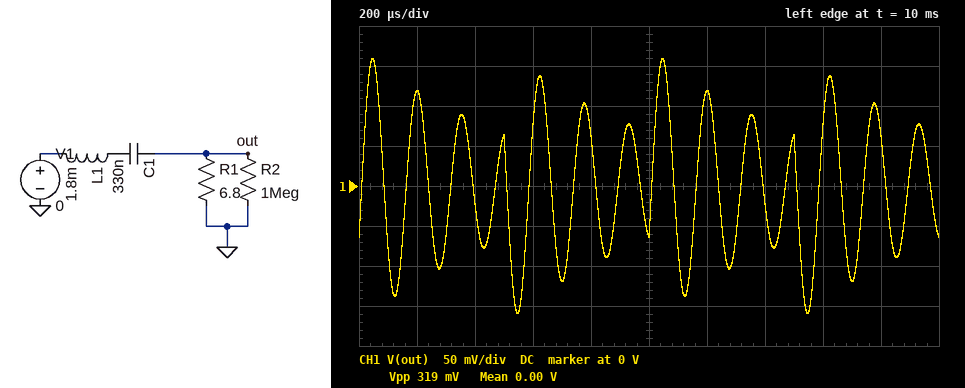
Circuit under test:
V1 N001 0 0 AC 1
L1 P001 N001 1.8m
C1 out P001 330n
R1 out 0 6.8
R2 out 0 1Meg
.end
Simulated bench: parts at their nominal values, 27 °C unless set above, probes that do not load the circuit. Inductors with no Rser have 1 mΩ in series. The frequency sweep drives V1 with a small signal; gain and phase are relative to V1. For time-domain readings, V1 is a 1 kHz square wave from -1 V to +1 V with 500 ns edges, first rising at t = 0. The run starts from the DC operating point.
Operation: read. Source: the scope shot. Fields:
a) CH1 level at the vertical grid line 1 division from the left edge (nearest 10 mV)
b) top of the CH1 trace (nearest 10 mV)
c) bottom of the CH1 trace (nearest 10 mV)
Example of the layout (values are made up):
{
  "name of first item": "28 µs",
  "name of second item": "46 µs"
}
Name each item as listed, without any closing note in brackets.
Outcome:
{
  "CH1 level at the vertical grid line 1 division from the left edge": "120 mV",
  "top of the CH1 trace": "160 mV",
  "bottom of the CH1 trace": "-160 mV"
}
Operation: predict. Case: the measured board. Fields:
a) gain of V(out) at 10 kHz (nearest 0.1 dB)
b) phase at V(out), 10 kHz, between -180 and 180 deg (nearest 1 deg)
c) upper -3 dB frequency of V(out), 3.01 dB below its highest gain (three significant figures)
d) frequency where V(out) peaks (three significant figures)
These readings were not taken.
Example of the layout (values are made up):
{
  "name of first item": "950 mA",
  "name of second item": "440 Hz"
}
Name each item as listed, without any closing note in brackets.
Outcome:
{
  "gain of V(out) at 10 kHz": "-19.6 dB",
  "phase at V(out), 10 kHz, between -180 and 180 deg": "-84 deg",
  "upper -3 dB frequency of V(out), 3.01 dB below its highest gain": "6.84 kHz",
  "frequency where V(out) peaks": "6.53 kHz"
}
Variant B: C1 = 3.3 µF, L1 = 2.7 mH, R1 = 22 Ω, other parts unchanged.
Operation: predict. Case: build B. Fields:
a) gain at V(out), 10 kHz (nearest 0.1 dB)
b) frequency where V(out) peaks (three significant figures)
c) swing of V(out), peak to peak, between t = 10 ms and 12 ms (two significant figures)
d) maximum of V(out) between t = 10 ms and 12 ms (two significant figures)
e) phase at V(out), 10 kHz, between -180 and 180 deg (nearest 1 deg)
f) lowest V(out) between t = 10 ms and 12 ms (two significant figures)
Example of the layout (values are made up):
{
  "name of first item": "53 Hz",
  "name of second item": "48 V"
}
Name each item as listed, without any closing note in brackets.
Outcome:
{
  "gain at V(out), 10 kHz": "-17.6 dB",
  "frequency where V(out) peaks": "1.69 kHz",
  "swing of V(out), peak to peak, between t = 10 ms and 12 ms": "1.9 V",
  "maximum of V(out) between t = 10 ms and 12 ms": "960 mV",
  "phase at V(out), 10 kHz, between -180 and 180 deg": "-82 deg",
  "lowest V(out) between t = 10 ms and 12 ms": "-960 mV"
}
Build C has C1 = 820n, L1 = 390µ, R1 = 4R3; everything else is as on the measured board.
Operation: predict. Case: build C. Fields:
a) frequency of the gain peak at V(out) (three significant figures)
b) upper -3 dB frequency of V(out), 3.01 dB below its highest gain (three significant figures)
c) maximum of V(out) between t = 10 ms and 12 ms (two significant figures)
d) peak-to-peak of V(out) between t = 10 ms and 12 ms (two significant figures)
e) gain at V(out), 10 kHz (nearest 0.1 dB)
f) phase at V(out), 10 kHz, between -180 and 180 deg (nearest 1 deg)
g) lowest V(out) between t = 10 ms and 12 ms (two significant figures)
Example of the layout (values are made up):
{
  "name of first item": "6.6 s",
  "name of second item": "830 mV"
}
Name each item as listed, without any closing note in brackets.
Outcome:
{
  "frequency of the gain peak at V(out)": "8.90 kHz",
  "upper -3 dB frequency of V(out), 3.01 dB below its highest gain": "9.82 kHz",
  "maximum of V(out) between t = 10 ms and 12 ms": "360 mV",
  "peak-to-peak of V(out) between t = 10 ms and 12 ms": "720 mV",
  "gain at V(out), 10 kHz": "-3.8 dB",
  "phase at V(out), 10 kHz, between -180 and 180 deg": "-50 deg",
  "lowest V(out) between t = 10 ms and 12 ms": "-360 mV"
}
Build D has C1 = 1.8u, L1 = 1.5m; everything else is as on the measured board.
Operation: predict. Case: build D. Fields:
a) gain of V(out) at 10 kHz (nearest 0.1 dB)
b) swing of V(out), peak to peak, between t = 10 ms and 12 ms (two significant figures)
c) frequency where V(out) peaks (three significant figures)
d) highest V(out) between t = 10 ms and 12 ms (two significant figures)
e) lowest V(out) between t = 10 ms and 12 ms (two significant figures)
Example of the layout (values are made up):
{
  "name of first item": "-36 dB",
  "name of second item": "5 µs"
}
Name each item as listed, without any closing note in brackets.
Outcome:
{
  "gain of V(out) at 10 kHz": "-22.0 dB",
  "swing of V(out), peak to peak, between t = 10 ms and 12 ms": "1.2 V",
  "frequency where V(out) peaks": "3.06 kHz",
  "highest V(out) between t = 10 ms and 12 ms": "590 mV",
  "lowest V(out) between t = 10 ms and 12 ms": "-590 mV"
}
